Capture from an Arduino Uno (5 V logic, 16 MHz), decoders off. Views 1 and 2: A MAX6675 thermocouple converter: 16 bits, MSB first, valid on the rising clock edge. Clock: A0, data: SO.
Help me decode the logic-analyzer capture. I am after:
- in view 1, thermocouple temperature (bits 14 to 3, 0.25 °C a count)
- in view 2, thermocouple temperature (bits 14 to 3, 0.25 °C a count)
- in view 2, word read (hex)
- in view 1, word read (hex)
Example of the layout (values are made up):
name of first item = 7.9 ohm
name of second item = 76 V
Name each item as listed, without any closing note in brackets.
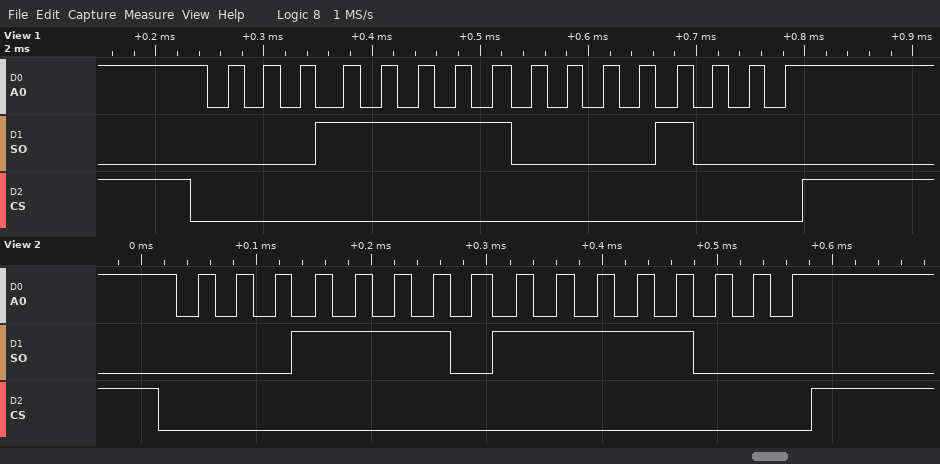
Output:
in view 1, thermocouple temperature = 248.25 °C
in view 2, thermocouple temperature = 247.75 °C
in view 2, word read = 0x1EF8
in view 1, word read = 0x1F08
